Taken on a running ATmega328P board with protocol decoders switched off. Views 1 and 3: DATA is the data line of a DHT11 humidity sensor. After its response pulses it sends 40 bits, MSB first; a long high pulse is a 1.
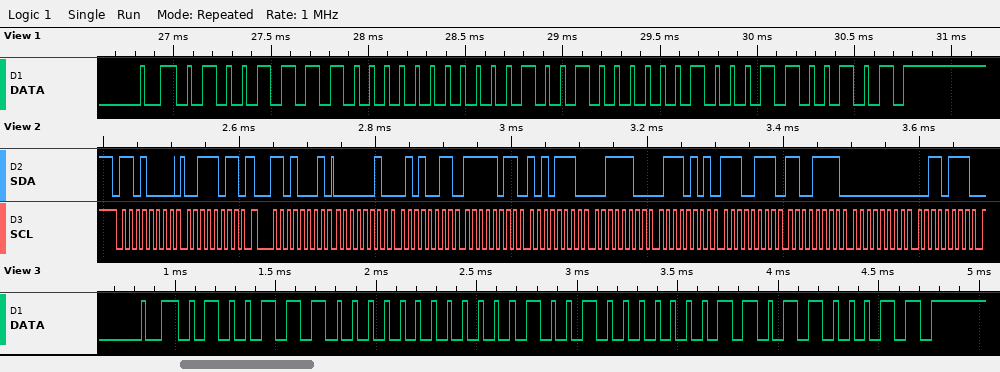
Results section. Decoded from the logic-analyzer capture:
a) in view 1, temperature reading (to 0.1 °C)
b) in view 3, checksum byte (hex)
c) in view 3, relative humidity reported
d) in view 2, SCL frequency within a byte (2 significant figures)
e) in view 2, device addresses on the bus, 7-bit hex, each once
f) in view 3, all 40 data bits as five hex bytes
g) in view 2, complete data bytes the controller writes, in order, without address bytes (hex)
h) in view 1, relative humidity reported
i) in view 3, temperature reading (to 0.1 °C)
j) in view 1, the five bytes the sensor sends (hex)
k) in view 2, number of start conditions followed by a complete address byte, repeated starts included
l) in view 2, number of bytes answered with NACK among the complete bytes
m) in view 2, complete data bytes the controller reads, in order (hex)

18.4 °C
0x63
78 %
100 kHz
0x68
4E 00 12 03 63
3B
79 %
18.3 °C
4F 00 12 04 65
2
0
02 53 FB AE 3C 75 E7 CF 00 37
